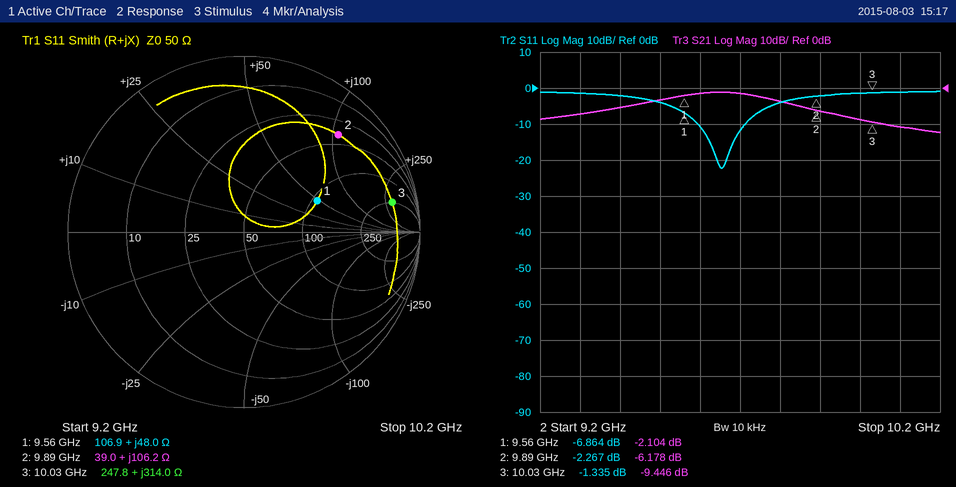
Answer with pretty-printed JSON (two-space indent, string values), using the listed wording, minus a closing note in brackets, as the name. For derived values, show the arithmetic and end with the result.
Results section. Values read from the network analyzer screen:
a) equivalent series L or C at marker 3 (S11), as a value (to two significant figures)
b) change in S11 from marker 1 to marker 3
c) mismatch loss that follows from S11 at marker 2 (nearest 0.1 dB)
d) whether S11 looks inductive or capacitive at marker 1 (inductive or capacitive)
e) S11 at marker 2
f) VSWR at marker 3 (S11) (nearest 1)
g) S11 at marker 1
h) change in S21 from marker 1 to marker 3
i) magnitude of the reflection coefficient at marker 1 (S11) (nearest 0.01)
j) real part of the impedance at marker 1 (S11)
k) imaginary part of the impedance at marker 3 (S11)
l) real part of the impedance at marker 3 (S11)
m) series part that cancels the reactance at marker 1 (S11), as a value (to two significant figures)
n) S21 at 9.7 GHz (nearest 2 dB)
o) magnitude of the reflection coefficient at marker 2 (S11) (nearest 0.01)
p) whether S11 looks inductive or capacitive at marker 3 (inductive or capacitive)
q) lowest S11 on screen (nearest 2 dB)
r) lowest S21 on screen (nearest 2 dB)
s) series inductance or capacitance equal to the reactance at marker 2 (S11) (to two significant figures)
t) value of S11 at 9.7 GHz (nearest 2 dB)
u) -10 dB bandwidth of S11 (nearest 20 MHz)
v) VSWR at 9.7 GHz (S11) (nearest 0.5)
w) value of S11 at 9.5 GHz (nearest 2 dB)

{
  "equivalent series L or C at marker 3 (S11), as a value": "L = 314 Ω/(2π × 10.03 GHz) ≈ 5.0 nH",
  "change in S11 from marker 1 to marker 3": "-1.335 − (-6.864) = 5.529 dB",
  "mismatch loss that follows from S11 at marker 2": "−10 log10(1 − 10^(-2.267/10)) ≈ 3.9 dB",
  "whether S11 looks inductive or capacitive at marker 1": "inductive",
  "S11 at marker 2": "-2.267 dB",
  "VSWR at marker 3 (S11)": "13",
  "S11 at marker 1": "-6.864 dB",
  "change in S21 from marker 1 to marker 3": "-9.446 − (-2.104) = -7.342 dB",
  "magnitude of the reflection coefficient at marker 1 (S11)": "0.45",
  "real part of the impedance at marker 1": "106.9 Ω",
  "imaginary part of the impedance at marker 3": "+314.0 Ω",
  "real part of the impedance at marker 3": "247.8 Ω",
  "series part that cancels the reactance at marker 1 (S11), as a value": "C = 1/(2π × 9.56 GHz × 48 Ω) ≈ 347 fF, so 350 fF to two significant figures",
  "S21 at 9.7 GHz": "-2 dB",
  "magnitude of the reflection coefficient at marker 2 (S11)": "0.77",
  "whether S11 looks inductive or capacitive at marker 3": "inductive",
  "lowest S11 on screen": "-22 dB",
  "lowest S21 on screen": "-12 dB",
  "series inductance or capacitance equal to the reactance at marker 2 (S11)": "L = 106.2 Ω/(2π × 9.89 GHz) ≈ 1.7 nH",
  "value of S11 at 9.7 GHz": "-12 dB",
  "-10 dB bandwidth of S11": "9.72 GHz − 9.60 GHz = 120 MHz",
  "VSWR at 9.7 GHz (S11)": "|Γ| = 10^(-12/20) = 0.2512; VSWR = (1 + 0.2512)/(1 − 0.2512) ≈ 1.67, so 1.5 to the nearest 0.5",
  "value of S11 at 9.5 GHz": "-4 dB"
}
